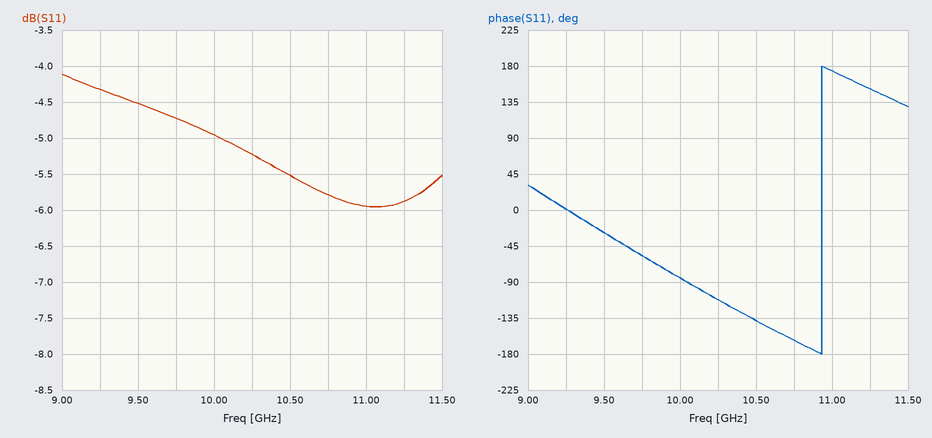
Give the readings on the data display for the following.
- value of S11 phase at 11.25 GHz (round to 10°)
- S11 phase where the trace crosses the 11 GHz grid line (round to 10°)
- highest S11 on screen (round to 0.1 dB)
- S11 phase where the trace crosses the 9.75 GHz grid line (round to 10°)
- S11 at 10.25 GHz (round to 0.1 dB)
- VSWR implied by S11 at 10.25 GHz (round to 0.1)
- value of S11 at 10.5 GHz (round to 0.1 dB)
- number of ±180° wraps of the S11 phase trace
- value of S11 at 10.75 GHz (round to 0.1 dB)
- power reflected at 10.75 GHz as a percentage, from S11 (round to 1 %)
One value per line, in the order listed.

150°
170°
-4.1 dB
-60°
-5.2 dB
3.4
-5.5 dB
1
-5.8 dB
26 %
